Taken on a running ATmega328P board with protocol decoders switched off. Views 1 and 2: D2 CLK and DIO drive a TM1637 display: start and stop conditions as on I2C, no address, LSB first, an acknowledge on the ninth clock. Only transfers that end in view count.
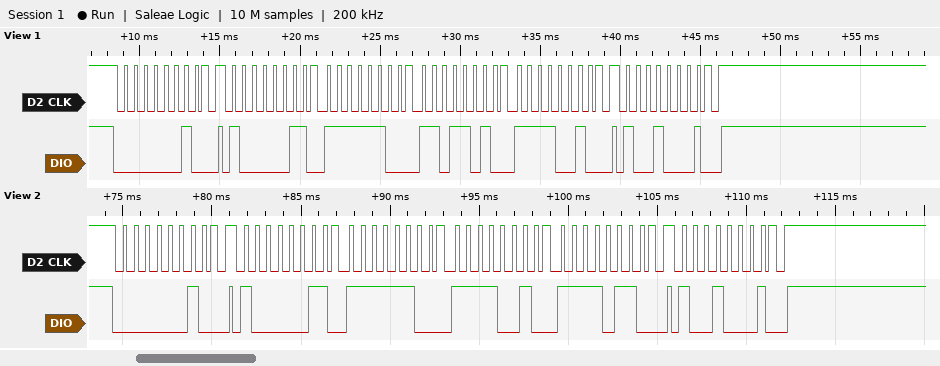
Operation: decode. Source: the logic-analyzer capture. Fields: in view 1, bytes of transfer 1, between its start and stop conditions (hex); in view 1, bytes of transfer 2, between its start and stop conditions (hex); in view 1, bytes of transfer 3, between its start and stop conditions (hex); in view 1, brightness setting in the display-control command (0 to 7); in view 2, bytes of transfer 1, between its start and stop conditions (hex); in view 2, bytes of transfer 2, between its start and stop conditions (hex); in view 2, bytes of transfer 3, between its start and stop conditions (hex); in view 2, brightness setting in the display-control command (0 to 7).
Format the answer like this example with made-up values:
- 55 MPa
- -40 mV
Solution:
- 40
- C1 3F 5B 4F
- 89
- 1
- 40
- C1 3F 4F 6F
- 89
- 1
